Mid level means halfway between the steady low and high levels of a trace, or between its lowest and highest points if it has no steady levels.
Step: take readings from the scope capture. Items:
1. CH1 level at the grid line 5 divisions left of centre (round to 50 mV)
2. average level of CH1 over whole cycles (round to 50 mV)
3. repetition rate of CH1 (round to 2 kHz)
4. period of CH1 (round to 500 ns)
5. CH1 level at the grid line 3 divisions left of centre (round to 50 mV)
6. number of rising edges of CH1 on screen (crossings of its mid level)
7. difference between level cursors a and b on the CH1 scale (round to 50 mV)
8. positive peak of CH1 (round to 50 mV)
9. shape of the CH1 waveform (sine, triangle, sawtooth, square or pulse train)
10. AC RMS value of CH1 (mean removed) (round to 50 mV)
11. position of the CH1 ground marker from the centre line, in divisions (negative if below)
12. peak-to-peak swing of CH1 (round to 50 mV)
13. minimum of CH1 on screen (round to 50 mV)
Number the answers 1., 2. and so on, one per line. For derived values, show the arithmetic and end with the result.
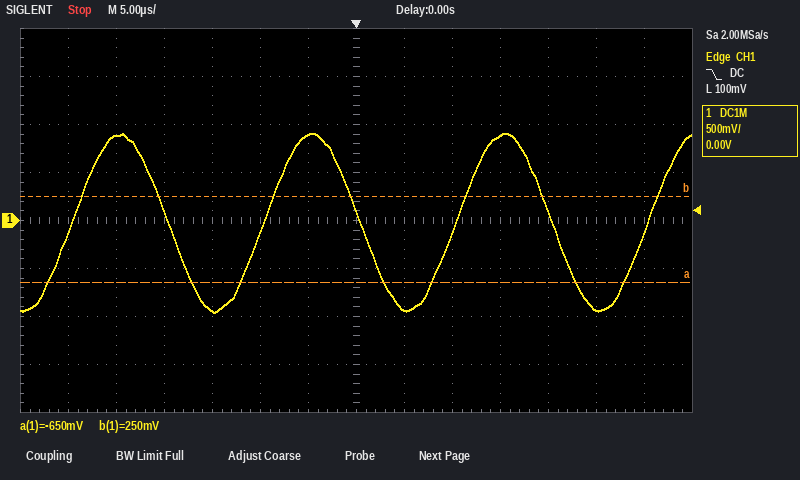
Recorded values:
1. 900 mV
2. (900 mV + (-950 mV)) / 2 ≈ 0 mV
3. 1 / 20.0 µs ≈ 50 kHz
4. 20.0 µs
5. -950 mV
6. 4
7. 900 mV
8. 900 mV
9. sine
10. 1.85 V / (2√2) ≈ 654 mV, so 650 mV to the nearest 50 mV
11. 0.0 div
12. 900 mV − (-950 mV) = 1.85 V
13. -950 mV
